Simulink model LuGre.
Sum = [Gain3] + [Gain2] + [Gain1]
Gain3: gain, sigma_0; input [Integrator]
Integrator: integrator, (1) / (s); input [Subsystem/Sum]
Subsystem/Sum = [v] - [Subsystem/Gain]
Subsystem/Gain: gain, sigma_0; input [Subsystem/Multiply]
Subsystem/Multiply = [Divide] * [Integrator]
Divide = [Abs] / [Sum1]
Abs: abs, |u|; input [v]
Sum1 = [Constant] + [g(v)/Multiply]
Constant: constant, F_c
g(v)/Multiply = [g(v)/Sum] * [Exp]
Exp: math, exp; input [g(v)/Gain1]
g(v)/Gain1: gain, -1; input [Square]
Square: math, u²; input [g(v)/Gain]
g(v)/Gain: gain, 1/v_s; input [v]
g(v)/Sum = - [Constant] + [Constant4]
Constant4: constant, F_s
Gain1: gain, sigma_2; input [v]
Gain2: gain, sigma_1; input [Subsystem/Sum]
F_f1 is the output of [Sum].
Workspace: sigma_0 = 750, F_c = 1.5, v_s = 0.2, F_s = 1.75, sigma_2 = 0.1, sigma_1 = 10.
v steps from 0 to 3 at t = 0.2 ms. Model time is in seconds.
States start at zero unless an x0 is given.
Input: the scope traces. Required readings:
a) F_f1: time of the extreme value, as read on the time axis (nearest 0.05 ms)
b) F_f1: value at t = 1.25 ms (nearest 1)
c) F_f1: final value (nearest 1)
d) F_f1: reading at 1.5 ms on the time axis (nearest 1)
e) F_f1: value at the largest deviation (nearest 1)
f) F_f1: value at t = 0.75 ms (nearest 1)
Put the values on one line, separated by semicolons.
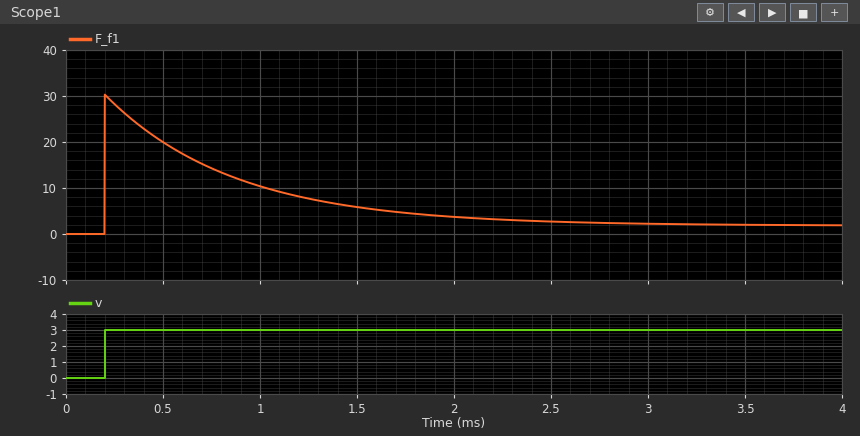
0.20 ms; 8; 2; 6; 30; 14
